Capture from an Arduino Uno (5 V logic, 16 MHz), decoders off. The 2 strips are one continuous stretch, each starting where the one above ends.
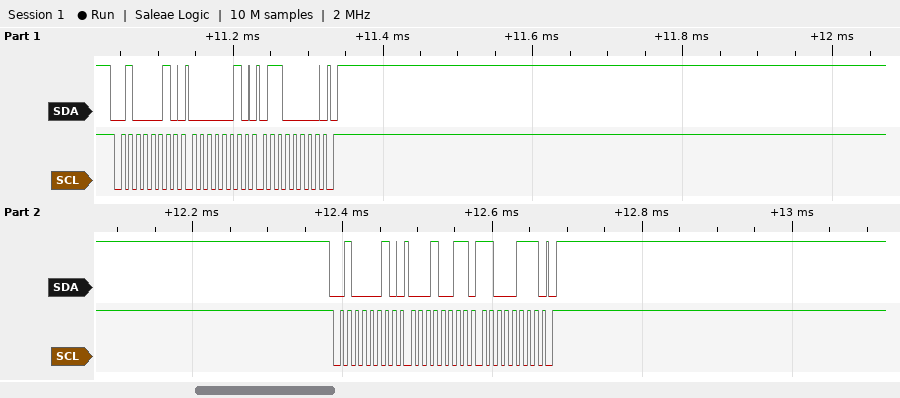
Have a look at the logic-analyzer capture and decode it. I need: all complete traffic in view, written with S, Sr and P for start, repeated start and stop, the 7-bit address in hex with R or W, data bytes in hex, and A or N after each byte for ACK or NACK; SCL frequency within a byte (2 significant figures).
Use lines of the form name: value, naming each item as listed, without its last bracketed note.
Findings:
all complete traffic in view, written with S, Sr and P for start, repeated start and stop, the 7-bit address in hex with R or W, data bytes in hex, and A or N after each byte for ACK or NACK: S 21W A 02 A 60 A P S 21W A 13 A C7 A P
SCL frequency within a byte: 100 kHz
